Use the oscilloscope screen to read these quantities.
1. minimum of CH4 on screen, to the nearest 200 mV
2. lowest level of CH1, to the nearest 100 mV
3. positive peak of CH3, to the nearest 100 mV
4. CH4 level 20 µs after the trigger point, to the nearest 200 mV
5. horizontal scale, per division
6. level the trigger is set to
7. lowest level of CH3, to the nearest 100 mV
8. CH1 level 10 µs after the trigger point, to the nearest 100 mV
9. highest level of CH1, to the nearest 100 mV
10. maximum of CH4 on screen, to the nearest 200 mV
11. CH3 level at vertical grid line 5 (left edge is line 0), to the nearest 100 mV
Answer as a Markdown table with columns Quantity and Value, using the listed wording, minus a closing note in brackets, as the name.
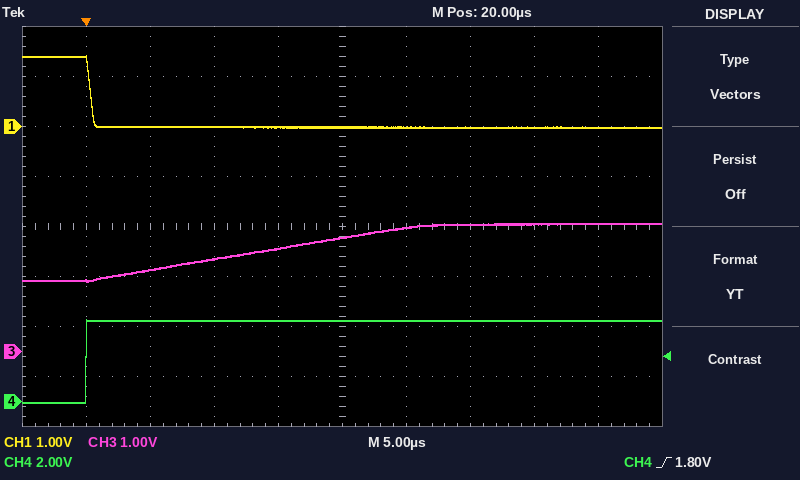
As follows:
| Quantity | Value |
|---|---|
| minimum of CH4 on screen, to the nearest 200 mV | 0.0 V |
| lowest level of CH1, to the nearest 100 mV | 0.0 V |
| positive peak of CH3, to the nearest 100 mV | 2.6 V |
| CH4 level 20 µs after the trigger point, to the nearest 200 mV | 3.2 V |
| horizontal scale, per division | 5 µs |
| level the trigger is set to | 1.80 V |
| lowest level of CH3, to the nearest 100 mV | 1.4 V |
| CH1 level 10 µs after the trigger point, to the nearest 100 mV | 0.0 V |
| highest level of CH1, to the nearest 100 mV | 1.4 V |
| maximum of CH4 on screen, to the nearest 200 mV | 3.2 V |
| CH3 level at vertical grid line 5 (left edge is line 0), to the nearest 100 mV | 2.3 V |
